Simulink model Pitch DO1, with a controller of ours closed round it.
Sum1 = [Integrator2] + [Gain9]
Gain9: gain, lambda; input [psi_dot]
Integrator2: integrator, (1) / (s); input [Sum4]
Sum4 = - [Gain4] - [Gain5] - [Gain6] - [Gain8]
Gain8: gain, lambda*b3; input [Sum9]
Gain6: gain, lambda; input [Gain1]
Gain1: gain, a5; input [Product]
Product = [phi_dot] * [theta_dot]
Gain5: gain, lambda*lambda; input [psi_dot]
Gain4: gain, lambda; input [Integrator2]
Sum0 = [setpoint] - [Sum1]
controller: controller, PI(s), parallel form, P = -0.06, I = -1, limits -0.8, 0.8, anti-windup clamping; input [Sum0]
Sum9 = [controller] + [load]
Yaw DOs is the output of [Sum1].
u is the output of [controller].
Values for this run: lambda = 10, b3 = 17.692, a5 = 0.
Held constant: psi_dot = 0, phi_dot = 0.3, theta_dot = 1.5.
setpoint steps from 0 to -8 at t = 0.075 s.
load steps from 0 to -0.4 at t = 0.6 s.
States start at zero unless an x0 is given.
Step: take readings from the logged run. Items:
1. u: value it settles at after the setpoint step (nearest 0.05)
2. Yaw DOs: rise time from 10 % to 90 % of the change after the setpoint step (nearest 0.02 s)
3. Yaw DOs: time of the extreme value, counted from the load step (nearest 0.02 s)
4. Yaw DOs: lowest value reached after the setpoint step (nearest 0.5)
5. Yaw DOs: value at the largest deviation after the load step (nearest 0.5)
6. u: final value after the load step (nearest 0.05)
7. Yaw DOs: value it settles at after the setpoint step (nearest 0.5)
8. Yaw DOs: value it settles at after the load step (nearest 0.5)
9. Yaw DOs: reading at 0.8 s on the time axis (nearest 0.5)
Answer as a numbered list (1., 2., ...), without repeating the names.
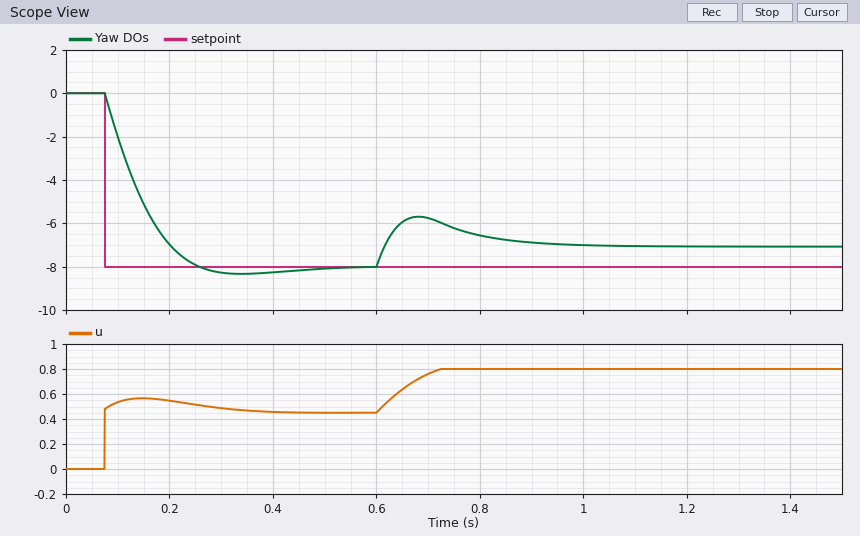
1. 0.45
2. 0.12 s
3. 0.08 s
4. -8.5
5. -5.5
6. 0.80
7. -8.0
8. -7.0
9. -6.5
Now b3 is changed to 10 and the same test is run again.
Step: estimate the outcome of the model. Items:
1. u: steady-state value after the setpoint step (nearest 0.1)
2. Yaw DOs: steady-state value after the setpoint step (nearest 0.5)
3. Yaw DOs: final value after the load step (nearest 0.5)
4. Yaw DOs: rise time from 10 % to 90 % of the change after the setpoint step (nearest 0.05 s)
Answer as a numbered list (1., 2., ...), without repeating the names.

1. 0.8
2. -8.0
3. -4.0
4. 0.25 s
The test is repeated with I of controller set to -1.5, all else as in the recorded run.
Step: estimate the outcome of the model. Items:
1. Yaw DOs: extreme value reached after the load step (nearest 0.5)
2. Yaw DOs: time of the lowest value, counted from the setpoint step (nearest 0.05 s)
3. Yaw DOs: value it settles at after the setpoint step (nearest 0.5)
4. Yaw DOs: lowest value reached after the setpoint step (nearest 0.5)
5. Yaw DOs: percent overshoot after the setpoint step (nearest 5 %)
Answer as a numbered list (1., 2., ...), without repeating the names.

1. -6.0
2. 0.20 s
3. -8.0
4. -9.0
5. 10 %
